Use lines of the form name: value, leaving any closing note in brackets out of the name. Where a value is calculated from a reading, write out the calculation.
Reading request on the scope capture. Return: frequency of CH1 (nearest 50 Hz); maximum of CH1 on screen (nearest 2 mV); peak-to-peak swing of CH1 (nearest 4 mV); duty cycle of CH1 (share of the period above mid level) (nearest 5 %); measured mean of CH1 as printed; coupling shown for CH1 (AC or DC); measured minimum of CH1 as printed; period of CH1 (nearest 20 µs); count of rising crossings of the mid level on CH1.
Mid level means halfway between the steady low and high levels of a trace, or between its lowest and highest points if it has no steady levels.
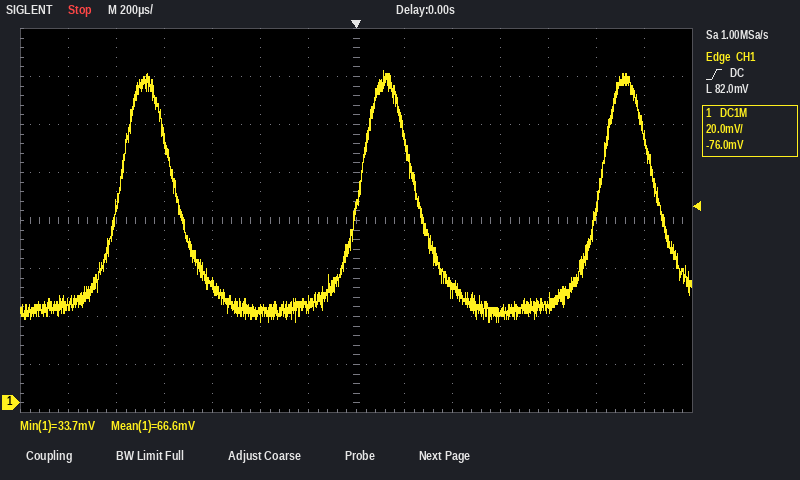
frequency of CH1: 1 / 1.00 ms ≈ 1.00 kHz
maximum of CH1 on screen: 138 mV
peak-to-peak swing of CH1: 104 mV
duty cycle of CH1 (share of the period above mid level): 25 %
measured mean of CH1 as printed: 66.6 mV
coupling shown for CH1: DC
measured minimum of CH1 as printed: 33.7 mV
period of CH1: 1.00 ms
count of rising crossings of the mid level on CH1: 3
